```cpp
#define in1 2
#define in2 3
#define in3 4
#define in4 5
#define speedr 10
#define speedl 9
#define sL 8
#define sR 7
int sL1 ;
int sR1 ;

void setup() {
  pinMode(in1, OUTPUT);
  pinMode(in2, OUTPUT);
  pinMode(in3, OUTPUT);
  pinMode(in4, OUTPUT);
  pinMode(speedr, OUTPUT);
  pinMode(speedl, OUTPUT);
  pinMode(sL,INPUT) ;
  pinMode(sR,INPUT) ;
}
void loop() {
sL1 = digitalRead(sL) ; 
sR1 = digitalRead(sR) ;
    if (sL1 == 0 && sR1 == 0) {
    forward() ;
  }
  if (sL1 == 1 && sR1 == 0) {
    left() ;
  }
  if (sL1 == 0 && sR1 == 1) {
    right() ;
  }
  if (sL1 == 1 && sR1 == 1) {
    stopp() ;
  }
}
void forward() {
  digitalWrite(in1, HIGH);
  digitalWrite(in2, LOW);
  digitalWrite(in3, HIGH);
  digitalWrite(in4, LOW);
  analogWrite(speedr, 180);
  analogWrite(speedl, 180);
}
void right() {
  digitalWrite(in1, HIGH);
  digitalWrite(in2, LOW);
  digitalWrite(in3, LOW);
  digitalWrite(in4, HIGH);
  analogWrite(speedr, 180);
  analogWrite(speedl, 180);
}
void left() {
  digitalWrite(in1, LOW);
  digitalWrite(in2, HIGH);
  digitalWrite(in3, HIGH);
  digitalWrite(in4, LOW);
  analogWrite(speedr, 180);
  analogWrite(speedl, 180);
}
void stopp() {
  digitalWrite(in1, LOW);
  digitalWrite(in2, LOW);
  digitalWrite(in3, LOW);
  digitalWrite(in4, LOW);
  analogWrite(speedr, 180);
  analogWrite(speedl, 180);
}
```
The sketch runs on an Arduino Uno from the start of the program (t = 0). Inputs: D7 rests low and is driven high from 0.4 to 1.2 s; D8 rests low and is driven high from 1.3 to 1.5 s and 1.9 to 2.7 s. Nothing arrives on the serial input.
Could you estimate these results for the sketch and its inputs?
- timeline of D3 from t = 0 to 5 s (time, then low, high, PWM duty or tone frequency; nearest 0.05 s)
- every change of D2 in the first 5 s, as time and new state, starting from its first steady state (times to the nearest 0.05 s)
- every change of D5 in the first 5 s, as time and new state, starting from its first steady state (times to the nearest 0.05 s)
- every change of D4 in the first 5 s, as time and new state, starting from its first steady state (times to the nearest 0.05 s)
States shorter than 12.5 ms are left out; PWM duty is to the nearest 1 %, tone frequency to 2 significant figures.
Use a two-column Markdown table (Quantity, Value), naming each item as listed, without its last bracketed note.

| Quantity | Value |
|---|---|
| timeline of D3 from t = 0 to 5 s | 0 s low; 1.3 s high; 1.5 s low; 1.9 s high; 2.7 s low |
| every change of D2 in the first 5 s, as time and new state, starting from its first steady state | 0 s high; 1.3 s low; 1.5 s high; 1.9 s low; 2.7 s high |
| every change of D5 in the first 5 s, as time and new state, starting from its first steady state | 0 s low; 0.4 s high; 1.2 s low |
| every change of D4 in the first 5 s, as time and new state, starting from its first steady state | 0 s high; 0.4 s low; 1.2 s high |
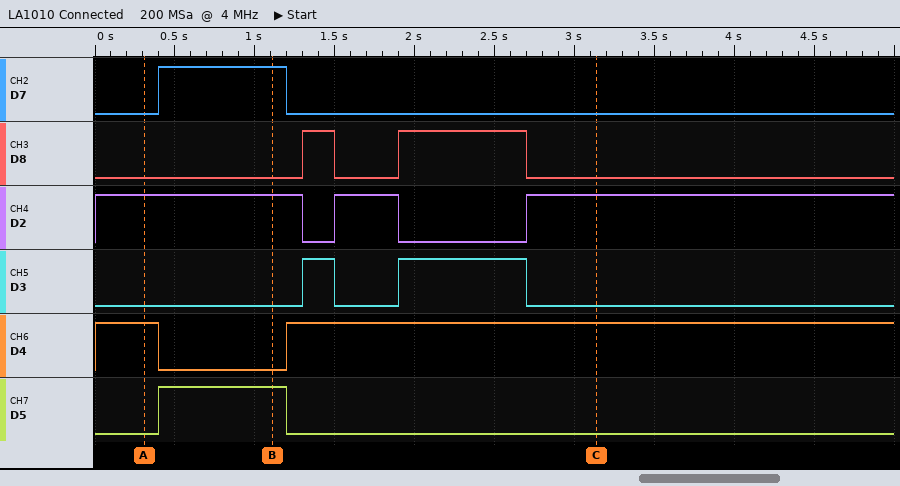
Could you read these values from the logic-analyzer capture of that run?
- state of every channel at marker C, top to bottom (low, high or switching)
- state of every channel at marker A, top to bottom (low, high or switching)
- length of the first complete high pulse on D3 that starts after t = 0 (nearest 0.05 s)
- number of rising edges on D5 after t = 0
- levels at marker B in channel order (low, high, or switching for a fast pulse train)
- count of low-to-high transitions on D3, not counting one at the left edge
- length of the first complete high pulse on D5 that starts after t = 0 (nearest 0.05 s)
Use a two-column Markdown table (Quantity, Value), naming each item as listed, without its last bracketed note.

| Quantity | Value |
|---|---|
| state of every channel at marker C, top to bottom | D7 low, D8 low, D2 high, D3 low, D4 high, D5 low |
| state of every channel at marker A, top to bottom | D7 low, D8 low, D2 high, D3 low, D4 high, D5 low |
| length of the first complete high pulse on D3 that starts after t = 0 | 0.20 s |
| number of rising edges on D5 after t = 0 | 1 |
| levels at marker B in channel order | D7 high, D8 low, D2 high, D3 low, D4 low, D5 high |
| count of low-to-high transitions on D3, not counting one at the left edge | 2 |
| length of the first complete high pulse on D5 that starts after t = 0 | 0.80 s |
